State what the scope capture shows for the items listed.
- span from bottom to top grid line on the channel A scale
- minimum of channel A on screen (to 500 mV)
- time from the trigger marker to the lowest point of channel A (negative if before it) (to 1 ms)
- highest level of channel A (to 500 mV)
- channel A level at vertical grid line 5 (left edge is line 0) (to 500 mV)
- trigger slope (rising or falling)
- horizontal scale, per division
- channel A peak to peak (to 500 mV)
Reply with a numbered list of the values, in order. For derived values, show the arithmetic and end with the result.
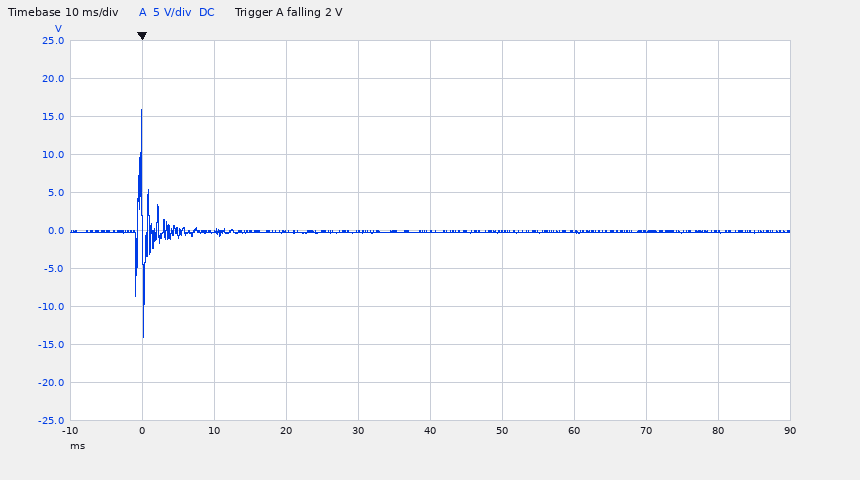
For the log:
1. 50 V
2. -14.0 V
3. 0 ms
4. 16.0 V
5. 0.0 V
6. falling
7. 10 ms
8. 16.0 V − (-14.0 V) = 30.0 V
